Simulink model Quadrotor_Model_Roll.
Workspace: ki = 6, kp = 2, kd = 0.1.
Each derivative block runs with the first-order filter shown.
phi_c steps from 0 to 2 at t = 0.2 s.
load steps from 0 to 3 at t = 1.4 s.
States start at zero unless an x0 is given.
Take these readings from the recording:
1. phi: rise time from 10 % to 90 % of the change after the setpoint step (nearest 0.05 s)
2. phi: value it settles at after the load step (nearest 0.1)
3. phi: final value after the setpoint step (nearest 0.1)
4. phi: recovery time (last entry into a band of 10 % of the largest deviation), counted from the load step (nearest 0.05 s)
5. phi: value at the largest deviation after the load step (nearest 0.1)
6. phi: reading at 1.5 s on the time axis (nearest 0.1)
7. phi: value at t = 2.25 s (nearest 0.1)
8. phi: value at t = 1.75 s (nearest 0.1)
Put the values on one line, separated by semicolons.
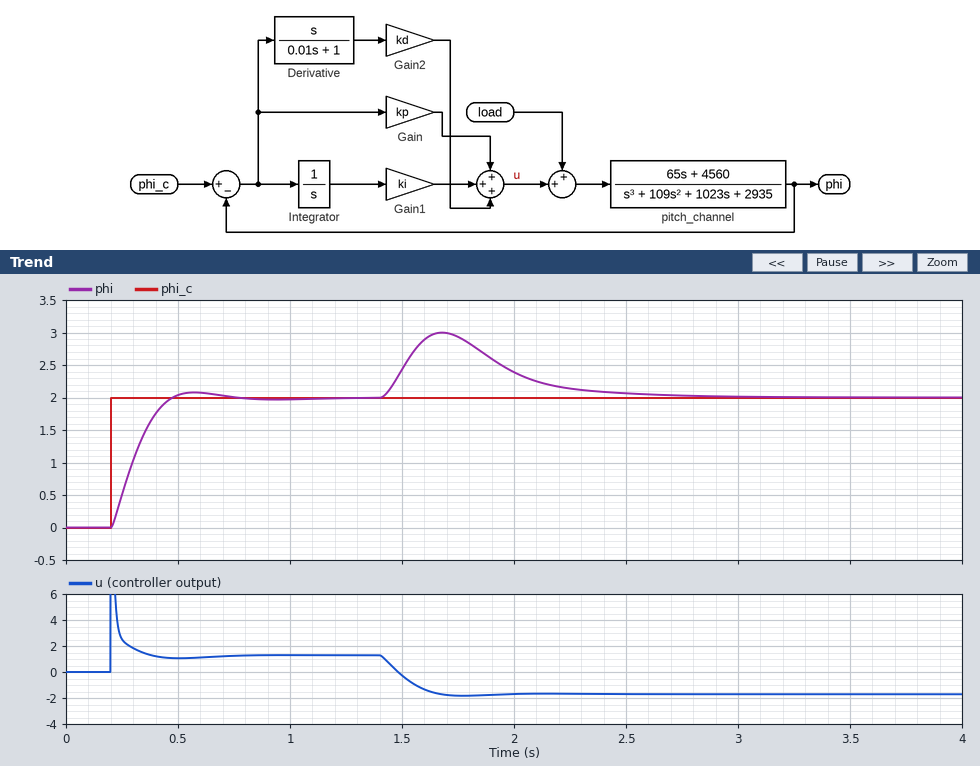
0.20 s; 2.0; 2.0; 0.95 s; 3.0; 2.4; 2.1; 2.9
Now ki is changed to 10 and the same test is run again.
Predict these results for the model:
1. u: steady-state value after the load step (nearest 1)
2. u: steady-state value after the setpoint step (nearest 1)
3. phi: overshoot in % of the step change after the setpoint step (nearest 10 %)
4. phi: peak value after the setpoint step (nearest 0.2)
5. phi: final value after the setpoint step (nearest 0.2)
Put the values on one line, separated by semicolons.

-2; 1; 20 %; 2.4; 2.0
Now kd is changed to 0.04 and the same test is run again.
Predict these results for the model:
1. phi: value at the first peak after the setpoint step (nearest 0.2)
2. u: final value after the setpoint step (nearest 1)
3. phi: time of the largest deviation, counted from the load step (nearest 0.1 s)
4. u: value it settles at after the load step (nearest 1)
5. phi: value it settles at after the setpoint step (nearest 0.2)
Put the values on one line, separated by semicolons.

2.2; 1; 0.3 s; -2; 2.0
